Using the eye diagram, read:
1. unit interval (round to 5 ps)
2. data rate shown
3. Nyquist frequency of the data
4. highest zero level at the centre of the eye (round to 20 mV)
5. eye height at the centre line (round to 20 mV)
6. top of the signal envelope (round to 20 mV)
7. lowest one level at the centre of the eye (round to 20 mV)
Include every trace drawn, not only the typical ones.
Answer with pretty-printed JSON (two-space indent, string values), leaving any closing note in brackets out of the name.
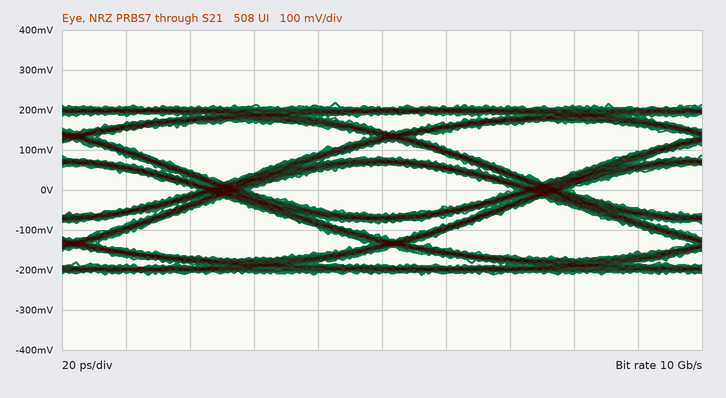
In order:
{
  "unit interval": "100 ps",
  "data rate shown": "10 Gb/s",
  "Nyquist frequency of the data": "5 GHz",
  "highest zero level at the centre of the eye": "-60 mV",
  "eye height at the centre line": "120 mV",
  "top of the signal envelope": "220 mV",
  "lowest one level at the centre of the eye": "60 mV"
}
